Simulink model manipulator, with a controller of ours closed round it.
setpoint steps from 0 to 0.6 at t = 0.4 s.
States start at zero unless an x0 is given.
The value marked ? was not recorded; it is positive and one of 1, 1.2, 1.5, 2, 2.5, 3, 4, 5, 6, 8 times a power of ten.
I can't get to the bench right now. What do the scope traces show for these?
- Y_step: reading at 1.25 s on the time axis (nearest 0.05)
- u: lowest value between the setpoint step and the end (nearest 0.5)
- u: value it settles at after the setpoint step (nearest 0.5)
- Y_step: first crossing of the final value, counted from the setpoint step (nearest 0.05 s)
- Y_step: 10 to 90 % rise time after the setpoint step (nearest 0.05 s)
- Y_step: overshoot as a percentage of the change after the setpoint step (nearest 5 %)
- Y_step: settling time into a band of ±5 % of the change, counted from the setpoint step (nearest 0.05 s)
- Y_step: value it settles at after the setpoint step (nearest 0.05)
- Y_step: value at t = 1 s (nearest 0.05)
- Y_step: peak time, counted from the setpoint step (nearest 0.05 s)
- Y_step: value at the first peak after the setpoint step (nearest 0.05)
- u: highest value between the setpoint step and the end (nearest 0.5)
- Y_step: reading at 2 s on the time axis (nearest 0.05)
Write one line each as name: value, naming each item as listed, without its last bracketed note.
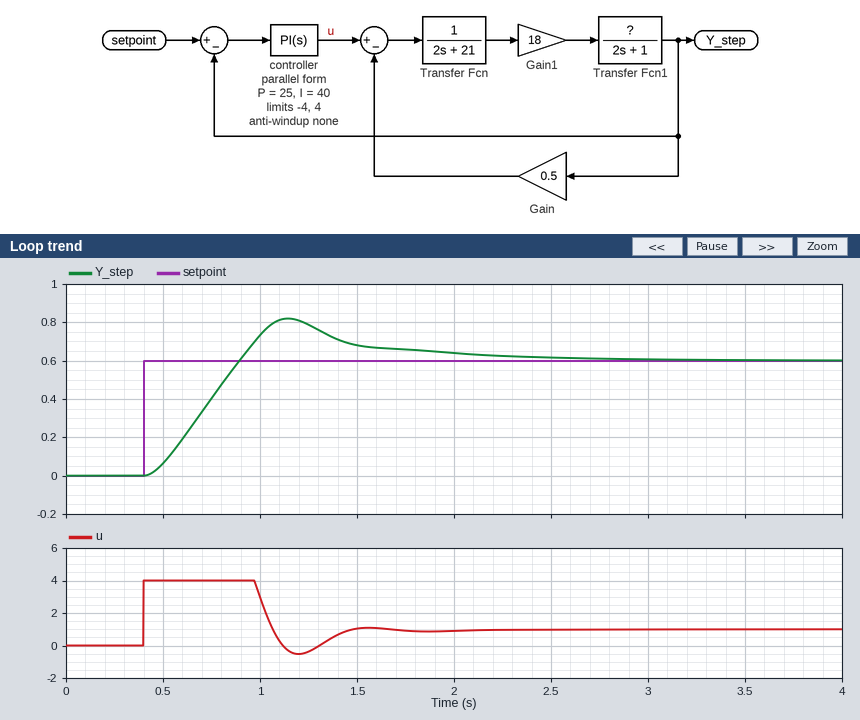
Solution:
Y_step: reading at 1.25 s on the time axis: 0.80
u: lowest value between the setpoint step and the end: -0.5
u: value it settles at after the setpoint step: 1.0
Y_step: first crossing of the final value, counted from the setpoint step: 0.50 s
Y_step: 10 to 90 % rise time after the setpoint step: 0.35 s
Y_step: overshoot as a percentage of the change after the setpoint step: 35 %
Y_step: settling time into a band of ±5 % of the change, counted from the setpoint step: 1.75 s
Y_step: value it settles at after the setpoint step: 0.60
Y_step: value at t = 1 s: 0.75
Y_step: peak time, counted from the setpoint step: 0.75 s
Y_step: value at the first peak after the setpoint step: 0.80
u: highest value between the setpoint step and the end: 4.0
Y_step: reading at 2 s on the time axis: 0.65
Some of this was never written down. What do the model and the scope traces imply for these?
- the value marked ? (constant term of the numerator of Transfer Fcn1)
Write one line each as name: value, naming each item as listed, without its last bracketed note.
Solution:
the value marked ?: 1
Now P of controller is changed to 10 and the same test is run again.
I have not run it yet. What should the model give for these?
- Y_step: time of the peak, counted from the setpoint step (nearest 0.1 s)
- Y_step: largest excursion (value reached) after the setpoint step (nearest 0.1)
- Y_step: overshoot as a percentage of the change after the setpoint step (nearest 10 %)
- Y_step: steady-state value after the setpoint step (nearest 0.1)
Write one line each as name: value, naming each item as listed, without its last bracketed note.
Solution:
Y_step: time of the peak, counted from the setpoint step: 0.9 s
Y_step: largest excursion (value reached) after the setpoint step: 0.9
Y_step: overshoot as a percentage of the change after the setpoint step: 60 %
Y_step: steady-state value after the setpoint step: 0.6
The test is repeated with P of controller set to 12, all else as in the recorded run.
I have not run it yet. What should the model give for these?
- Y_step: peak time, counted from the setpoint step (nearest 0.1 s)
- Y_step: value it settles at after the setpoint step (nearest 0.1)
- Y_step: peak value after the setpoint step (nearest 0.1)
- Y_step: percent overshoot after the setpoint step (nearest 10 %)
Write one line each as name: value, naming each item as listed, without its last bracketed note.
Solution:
Y_step: peak time, counted from the setpoint step: 0.8 s
Y_step: value it settles at after the setpoint step: 0.6
Y_step: peak value after the setpoint step: 0.9
Y_step: percent overshoot after the setpoint step: 50 %
